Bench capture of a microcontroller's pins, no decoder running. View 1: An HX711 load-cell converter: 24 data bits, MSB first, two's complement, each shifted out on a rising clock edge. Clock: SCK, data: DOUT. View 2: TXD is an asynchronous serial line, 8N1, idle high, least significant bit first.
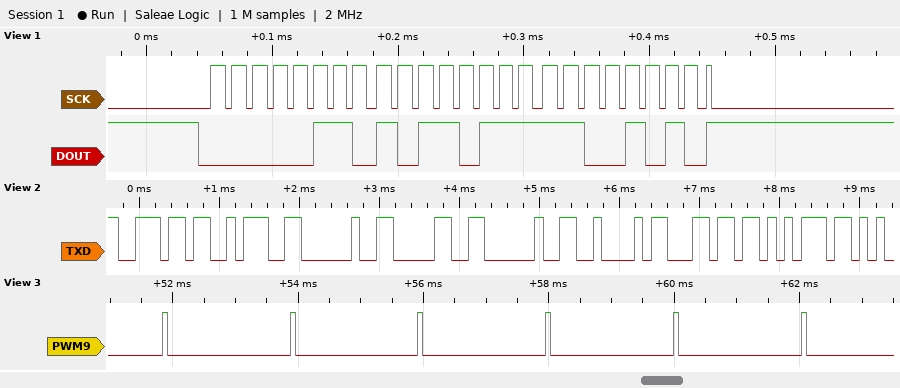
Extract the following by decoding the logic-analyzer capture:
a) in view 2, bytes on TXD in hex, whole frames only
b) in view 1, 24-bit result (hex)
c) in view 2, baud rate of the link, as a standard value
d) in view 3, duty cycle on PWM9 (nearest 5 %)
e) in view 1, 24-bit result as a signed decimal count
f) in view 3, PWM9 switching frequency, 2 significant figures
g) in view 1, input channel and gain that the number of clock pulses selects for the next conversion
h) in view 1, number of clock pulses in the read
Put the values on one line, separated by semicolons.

6E 3A 20 30 20 42 6C 75; 0x06B7CA; 9600 baud; 5 %; 440266; 490 Hz; channel A, gain 128; 25
